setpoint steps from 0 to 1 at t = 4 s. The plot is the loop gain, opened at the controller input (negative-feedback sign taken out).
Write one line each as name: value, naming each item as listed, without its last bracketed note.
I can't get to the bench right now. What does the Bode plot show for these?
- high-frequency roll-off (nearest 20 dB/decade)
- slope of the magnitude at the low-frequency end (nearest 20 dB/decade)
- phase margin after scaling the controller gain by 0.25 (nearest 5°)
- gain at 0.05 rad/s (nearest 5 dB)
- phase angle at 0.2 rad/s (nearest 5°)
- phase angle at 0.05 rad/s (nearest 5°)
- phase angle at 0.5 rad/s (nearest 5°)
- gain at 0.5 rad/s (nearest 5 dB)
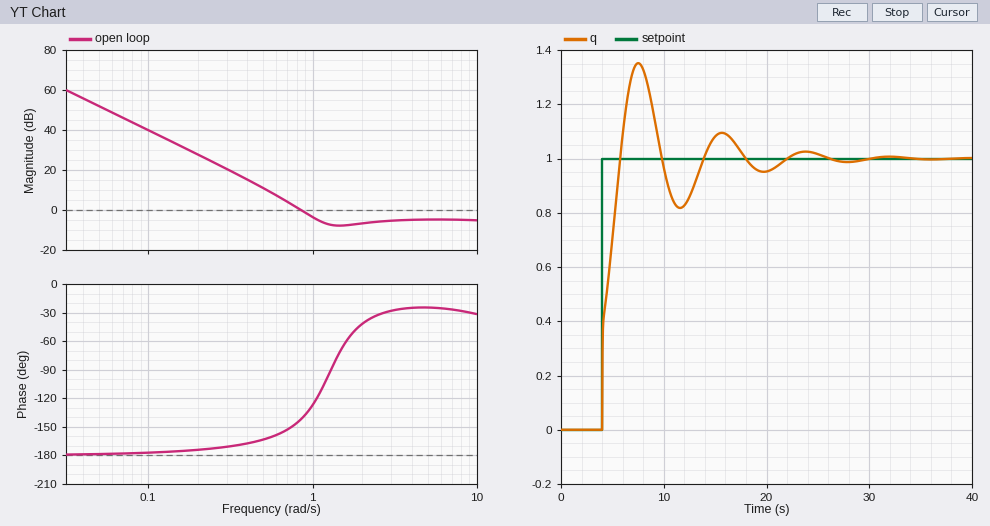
high-frequency roll-off: 0 dB/decade
slope of the magnitude at the low-frequency end: -40 dB/decade
phase margin after scaling the controller gain by 0.25: 15°
gain at 0.05 rad/s: 50 dB
phase angle at 0.2 rad/s: -175°
phase angle at 0.05 rad/s: -180°
phase angle at 0.5 rad/s: -165°
gain at 0.5 rad/s: 10 dB
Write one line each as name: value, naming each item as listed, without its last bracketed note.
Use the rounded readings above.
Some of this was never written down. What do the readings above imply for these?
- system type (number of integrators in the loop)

system type: 2
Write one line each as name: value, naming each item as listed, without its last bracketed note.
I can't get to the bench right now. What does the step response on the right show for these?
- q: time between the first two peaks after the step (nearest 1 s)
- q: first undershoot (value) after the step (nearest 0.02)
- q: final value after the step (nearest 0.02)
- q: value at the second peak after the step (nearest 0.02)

q: time between the first two peaks after the step: 8 s
q: first undershoot (value) after the step: 0.82
q: final value after the step: 1.00
q: value at the second peak after the step: 1.10
